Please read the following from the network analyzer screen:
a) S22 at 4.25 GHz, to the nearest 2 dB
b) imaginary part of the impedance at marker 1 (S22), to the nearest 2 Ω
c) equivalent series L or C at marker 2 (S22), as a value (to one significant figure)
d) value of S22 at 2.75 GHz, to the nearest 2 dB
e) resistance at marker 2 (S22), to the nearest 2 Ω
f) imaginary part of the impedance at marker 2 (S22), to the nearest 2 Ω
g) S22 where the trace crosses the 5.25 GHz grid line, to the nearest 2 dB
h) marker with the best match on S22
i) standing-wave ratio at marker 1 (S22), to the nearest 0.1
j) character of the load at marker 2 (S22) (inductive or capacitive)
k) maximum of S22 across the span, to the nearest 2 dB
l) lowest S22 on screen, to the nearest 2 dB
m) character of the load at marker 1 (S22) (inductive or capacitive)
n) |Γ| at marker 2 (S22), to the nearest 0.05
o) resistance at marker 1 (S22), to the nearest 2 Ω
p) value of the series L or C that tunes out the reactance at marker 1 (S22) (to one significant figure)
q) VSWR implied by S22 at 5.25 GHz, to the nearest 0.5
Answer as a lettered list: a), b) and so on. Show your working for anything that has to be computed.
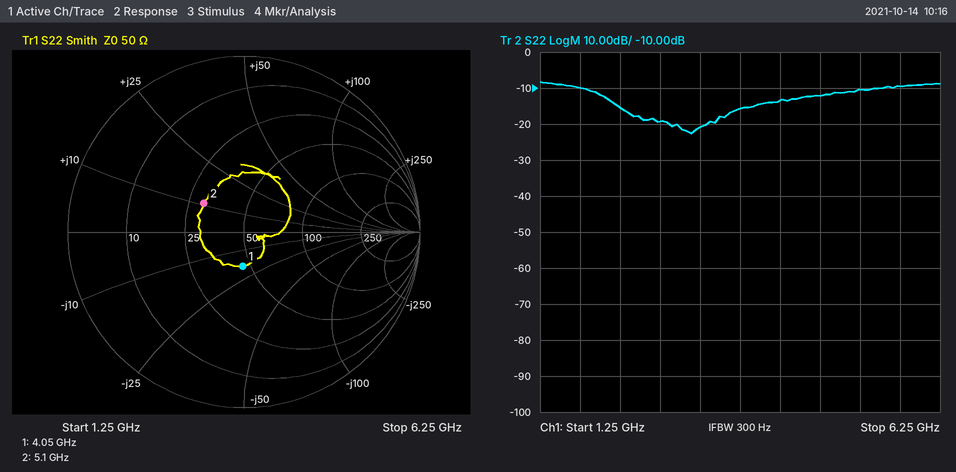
a) -14 dB
b) -18 Ω
c) L = 10 Ω/(2π × 5.1 GHz) ≈ 312 pH, so 300 pH to one significant figure
d) -20 dB
e) 30 Ω
f) +10 Ω
g) -10 dB
h) marker 1
i) 1.5
j) inductive
k) -8 dB
l) -22 dB
m) capacitive
n) 0.30
o) 46 Ω
p) L = 18 Ω/(2π × 4.05 GHz) ≈ 707 pH, so 700 pH to one significant figure
q) |Γ| = 10^(-10/20) = 0.3162; VSWR = (1 + 0.3162)/(1 − 0.3162) ≈ 1.92, so 2.0 to the nearest 0.5
